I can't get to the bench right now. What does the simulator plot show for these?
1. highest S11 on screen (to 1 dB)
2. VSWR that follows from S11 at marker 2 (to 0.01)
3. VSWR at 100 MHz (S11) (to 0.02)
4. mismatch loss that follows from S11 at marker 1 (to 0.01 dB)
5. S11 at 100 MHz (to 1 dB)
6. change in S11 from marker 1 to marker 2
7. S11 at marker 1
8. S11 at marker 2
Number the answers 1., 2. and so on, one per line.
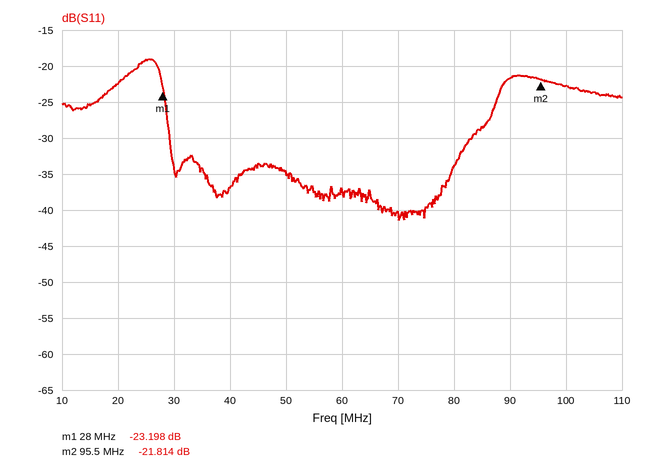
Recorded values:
1. -19 dB
2. 1.18
3. 1.16
4. 0.02 dB
5. -23 dB
6. 1.384 dB
7. -23.198 dB
8. -21.814 dB
